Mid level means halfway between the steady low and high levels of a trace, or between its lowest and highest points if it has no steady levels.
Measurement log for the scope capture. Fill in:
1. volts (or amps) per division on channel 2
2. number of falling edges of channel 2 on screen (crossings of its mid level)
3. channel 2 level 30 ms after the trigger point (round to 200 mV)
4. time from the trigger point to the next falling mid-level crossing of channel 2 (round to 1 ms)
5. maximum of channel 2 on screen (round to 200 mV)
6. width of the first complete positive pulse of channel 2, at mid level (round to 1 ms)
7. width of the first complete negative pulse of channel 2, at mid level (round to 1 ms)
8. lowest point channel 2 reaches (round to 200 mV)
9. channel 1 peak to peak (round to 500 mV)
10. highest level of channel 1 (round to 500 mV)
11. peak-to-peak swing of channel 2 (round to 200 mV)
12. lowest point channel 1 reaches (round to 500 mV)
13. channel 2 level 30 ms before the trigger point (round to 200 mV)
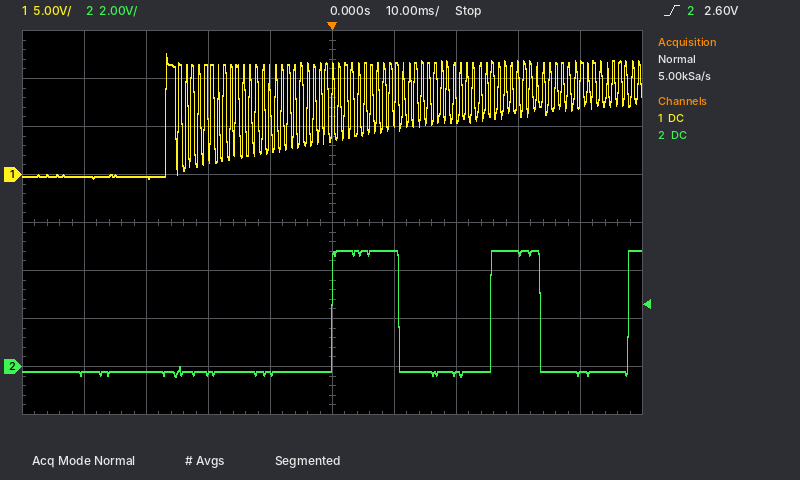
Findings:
2 V
2
4.8 V
11 ms
4.8 V
11 ms
15 ms
-400 mV
13.0 V
12.5 V
5.2 V
-500 mV
-200 mV
